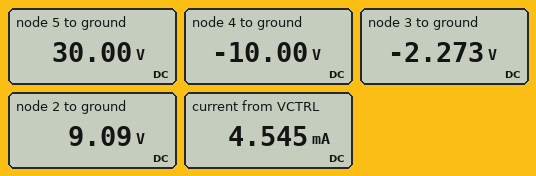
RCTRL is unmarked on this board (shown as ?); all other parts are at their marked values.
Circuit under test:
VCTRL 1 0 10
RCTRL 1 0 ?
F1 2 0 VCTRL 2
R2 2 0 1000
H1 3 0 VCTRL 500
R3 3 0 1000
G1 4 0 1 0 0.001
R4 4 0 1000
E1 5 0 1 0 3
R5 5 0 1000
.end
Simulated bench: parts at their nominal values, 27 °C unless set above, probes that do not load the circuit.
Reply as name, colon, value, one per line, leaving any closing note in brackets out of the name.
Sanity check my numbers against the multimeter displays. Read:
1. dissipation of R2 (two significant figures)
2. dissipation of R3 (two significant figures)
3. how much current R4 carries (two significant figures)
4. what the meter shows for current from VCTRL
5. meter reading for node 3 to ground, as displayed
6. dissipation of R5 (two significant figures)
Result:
dissipation of R2: 83 mW
dissipation of R3: 5.2 mW
how much current R4 carries: 10 mA
what the meter shows for current from VCTRL: 4.545 mA
meter reading for node 3 to ground, as displayed: -2.273 V
dissipation of R5: 900 mW
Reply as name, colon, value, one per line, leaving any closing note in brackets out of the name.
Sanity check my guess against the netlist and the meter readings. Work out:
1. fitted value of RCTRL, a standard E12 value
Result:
fitted value of RCTRL, a standard E12 value: 2.2 kΩ
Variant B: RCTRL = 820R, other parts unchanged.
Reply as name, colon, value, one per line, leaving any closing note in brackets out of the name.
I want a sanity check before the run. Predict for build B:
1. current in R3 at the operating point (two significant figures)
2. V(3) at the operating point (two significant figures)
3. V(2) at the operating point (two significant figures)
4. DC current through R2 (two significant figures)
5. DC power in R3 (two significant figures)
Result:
current in R3 at the operating point: 6.1 mA
V(3) at the operating point: -6.1 V
V(2) at the operating point: 24 V
DC current through R2: 24 mA
DC power in R3: 37 mW
